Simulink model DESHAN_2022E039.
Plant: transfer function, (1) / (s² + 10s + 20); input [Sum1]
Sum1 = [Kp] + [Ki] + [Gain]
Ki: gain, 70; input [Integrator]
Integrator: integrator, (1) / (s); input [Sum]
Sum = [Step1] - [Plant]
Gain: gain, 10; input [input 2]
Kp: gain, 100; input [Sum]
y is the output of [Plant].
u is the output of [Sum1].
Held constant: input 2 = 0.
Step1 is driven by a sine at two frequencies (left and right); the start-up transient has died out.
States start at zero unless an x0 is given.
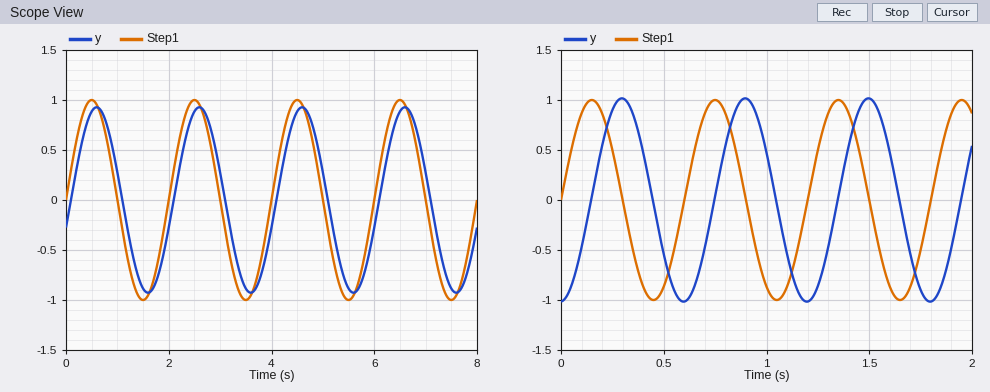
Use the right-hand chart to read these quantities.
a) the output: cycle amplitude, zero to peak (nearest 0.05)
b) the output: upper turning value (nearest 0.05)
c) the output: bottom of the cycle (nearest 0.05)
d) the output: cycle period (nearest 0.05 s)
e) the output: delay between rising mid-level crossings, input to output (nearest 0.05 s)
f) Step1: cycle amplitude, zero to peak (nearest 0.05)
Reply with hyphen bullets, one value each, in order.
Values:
- 1.00
- 1.00
- -1.00
- 0.60 s
- 0.15 s
- 1.00
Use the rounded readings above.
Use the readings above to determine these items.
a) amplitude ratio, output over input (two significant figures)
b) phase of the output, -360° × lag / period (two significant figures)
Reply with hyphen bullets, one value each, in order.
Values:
- 1.0
- -90°
